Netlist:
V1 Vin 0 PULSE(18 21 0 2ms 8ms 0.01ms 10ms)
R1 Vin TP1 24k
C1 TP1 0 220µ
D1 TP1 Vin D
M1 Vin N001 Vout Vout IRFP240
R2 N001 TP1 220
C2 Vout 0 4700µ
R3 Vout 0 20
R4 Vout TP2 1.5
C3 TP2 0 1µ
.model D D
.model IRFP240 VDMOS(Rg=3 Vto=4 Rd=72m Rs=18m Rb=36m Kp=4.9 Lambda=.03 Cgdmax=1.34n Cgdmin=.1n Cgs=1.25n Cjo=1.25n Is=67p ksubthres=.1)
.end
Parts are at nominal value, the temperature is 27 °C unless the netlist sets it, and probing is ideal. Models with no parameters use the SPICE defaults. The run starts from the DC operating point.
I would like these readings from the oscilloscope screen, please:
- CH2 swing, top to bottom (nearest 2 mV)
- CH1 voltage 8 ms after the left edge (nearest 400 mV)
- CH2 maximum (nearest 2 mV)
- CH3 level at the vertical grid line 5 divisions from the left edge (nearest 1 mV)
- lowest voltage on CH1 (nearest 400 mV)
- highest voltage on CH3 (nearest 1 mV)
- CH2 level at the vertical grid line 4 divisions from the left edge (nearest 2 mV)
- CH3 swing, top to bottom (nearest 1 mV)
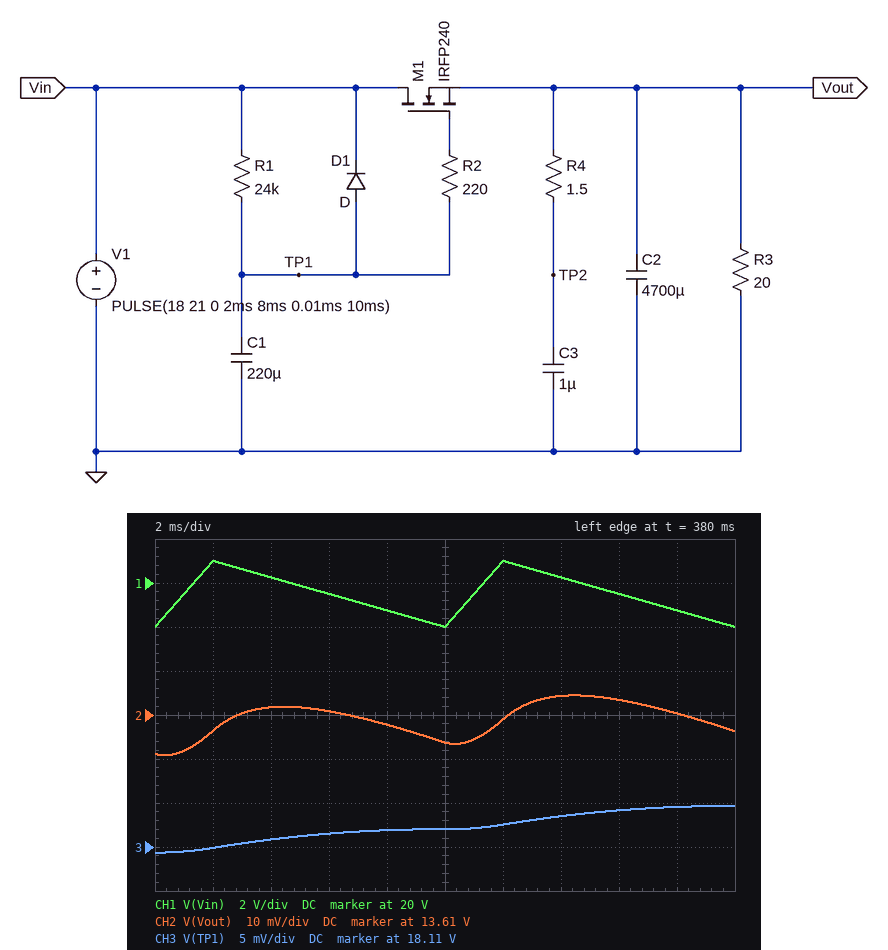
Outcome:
14 mV
18.8 V
13.614 V
18.107 V
18.0 V
18.110 V
13.608 V
5 mV
